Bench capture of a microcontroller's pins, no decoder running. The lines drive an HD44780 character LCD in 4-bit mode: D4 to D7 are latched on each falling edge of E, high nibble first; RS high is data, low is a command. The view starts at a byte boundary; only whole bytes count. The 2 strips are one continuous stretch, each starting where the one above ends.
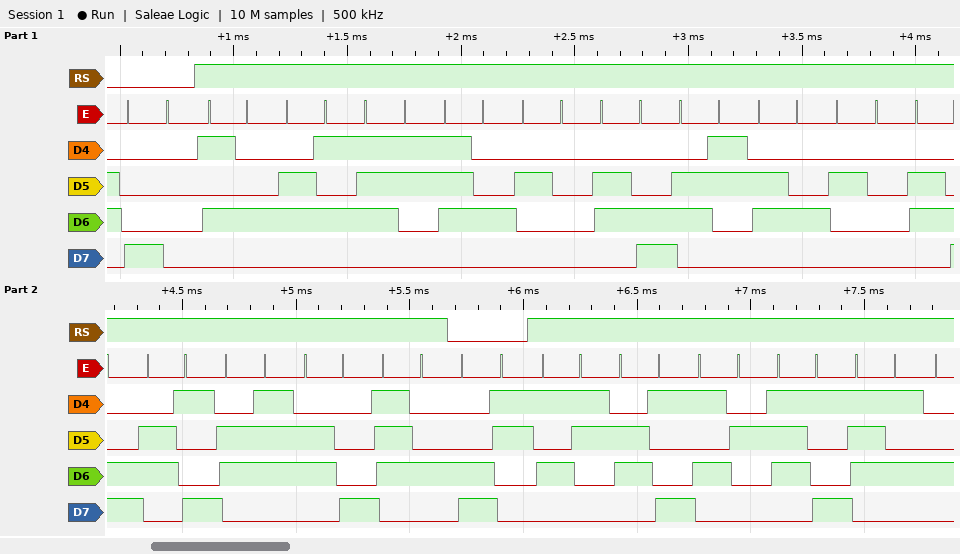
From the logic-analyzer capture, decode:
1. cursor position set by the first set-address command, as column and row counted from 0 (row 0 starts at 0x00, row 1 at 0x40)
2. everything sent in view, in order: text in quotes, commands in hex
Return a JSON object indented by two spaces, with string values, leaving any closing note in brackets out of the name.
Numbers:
{
  "cursor position set by the first set-address command, as column and row counted from 0": "column 0, row 0",
  "everything sent in view, in order: text in quotes, commands in hex": "0x80 \"Test lcd light\" 0xC3 \"SiRyu\""
}
